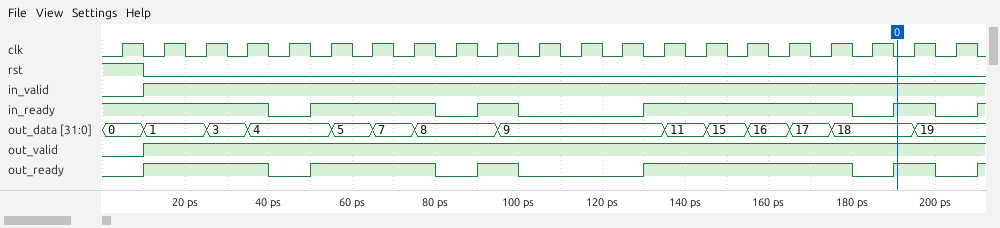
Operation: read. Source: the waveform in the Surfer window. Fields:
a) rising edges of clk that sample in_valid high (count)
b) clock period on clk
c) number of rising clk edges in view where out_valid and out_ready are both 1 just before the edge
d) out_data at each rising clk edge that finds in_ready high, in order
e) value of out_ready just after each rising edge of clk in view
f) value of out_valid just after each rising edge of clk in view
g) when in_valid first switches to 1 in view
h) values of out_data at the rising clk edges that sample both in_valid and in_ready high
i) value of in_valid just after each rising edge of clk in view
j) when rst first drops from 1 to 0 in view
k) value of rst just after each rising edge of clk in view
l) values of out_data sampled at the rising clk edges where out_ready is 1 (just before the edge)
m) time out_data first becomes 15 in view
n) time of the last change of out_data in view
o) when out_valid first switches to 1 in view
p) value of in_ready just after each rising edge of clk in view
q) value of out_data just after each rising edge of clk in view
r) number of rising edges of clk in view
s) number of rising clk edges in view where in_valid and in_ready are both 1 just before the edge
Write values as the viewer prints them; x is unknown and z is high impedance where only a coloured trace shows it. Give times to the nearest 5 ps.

20
10 ps
13
0, 1, 1, 3, 4, 5, 7, 8, 9, 11, 15, 16, 17, 18
0 1 1 1 0 1 1 1 0 1 0 0 0 1 1 1 1 1 0 1 0
0 1 1 1 1 1 1 1 1 1 1 1 1 1 1 1 1 1 1 1 1
10 ps
1, 1, 3, 4, 5, 7, 8, 9, 11, 15, 16, 17, 18
0 1 1 1 1 1 1 1 1 1 1 1 1 1 1 1 1 1 1 1 1
10 ps
1 0 0 0 0 0 0 0 0 0 0 0 0 0 0 0 0 0 0 0 0
1, 1, 3, 4, 5, 7, 8, 9, 11, 15, 16, 17, 18
145 ps
195 ps
10 ps
1 1 1 1 0 1 1 1 0 1 0 0 0 1 1 1 1 1 0 1 0
0, 1, 3, 4, 4, 5, 7, 8, 8, 9, 9, 9, 9, 11, 15, 16, 17, 18, 18, 19, 19
21
13
